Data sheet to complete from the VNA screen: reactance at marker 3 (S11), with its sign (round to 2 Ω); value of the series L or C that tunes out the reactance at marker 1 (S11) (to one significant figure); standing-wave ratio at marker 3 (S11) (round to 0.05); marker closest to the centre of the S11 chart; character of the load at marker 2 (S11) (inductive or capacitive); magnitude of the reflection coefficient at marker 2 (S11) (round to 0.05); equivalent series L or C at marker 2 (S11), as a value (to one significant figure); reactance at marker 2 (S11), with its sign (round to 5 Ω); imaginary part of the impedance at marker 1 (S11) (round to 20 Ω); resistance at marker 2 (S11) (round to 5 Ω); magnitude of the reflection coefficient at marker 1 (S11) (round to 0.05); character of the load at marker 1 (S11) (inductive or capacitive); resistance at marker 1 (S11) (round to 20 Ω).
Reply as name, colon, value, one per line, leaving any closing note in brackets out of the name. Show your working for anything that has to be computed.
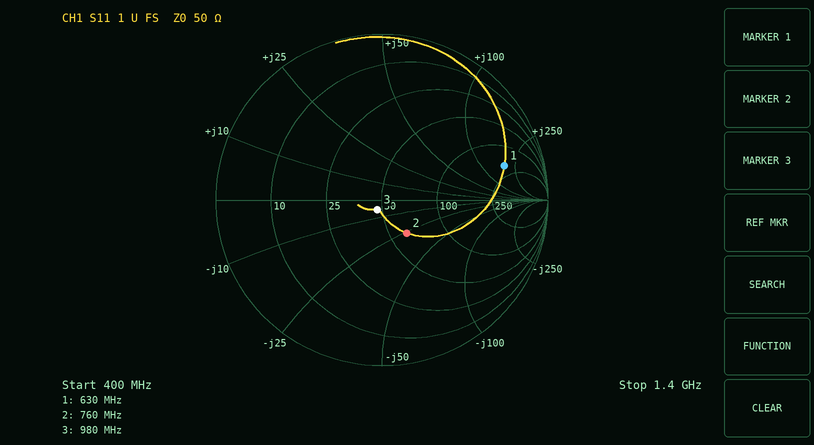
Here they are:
reactance at marker 3 (S11), with its sign: -6 Ω
value of the series L or C that tunes out the reactance at marker 1 (S11): C = 1/(2π × 630 MHz × 180 Ω) ≈ 1 pF
standing-wave ratio at marker 3 (S11): 1.15
marker closest to the centre of the S11 chart: marker 3
character of the load at marker 2 (S11): capacitive
magnitude of the reflection coefficient at marker 2 (S11): 0.25
equivalent series L or C at marker 2 (S11), as a value: C = 1/(2π × 760 MHz × 25 Ω) ≈ 8 pF
reactance at marker 2 (S11), with its sign: -25 Ω
imaginary part of the impedance at marker 1 (S11): +180 Ω
resistance at marker 2 (S11): 60 Ω
magnitude of the reflection coefficient at marker 1 (S11): 0.75
character of the load at marker 1 (S11): inductive
resistance at marker 1 (S11): 180 Ω
